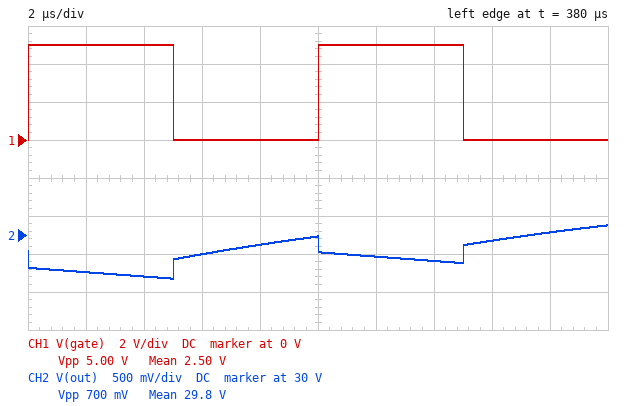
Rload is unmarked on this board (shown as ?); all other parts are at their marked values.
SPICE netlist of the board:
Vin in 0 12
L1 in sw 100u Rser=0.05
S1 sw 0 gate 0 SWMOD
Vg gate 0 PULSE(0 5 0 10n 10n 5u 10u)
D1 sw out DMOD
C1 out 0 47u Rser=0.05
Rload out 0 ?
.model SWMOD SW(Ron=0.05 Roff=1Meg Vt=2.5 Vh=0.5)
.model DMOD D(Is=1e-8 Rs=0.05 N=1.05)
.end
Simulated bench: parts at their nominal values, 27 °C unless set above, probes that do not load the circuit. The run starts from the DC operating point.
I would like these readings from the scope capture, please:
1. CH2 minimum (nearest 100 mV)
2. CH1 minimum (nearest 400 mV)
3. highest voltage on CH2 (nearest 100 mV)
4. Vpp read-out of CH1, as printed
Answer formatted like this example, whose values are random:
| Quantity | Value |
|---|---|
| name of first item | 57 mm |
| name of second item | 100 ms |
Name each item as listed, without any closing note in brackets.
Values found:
| Quantity | Value |
|---|---|
| CH2 minimum | 29.4 V |
| CH1 minimum | 0 V |
| highest voltage on CH2 | 30.1 V |
| Vpp read-out of CH1, as printed | 5.00 V |
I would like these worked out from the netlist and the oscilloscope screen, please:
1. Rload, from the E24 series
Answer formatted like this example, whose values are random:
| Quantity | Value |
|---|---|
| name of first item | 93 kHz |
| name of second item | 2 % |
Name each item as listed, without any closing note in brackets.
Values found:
| Quantity | Value |
|---|---|
| Rload, from the E24 series | 22 Ω |
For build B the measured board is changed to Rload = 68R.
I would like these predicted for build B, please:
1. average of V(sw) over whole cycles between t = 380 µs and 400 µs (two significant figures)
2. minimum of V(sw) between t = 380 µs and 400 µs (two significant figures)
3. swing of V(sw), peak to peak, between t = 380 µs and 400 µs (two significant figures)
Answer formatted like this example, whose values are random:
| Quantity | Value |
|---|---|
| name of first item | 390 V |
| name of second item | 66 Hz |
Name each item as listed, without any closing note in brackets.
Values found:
| Quantity | Value |
|---|---|
| average of V(sw) over whole cycles between t = 380 µs and 400 µs | 16 V |
| minimum of V(sw) between t = 380 µs and 400 µs | 120 mV |
| swing of V(sw), peak to peak, between t = 380 µs and 400 µs | 32 V |
